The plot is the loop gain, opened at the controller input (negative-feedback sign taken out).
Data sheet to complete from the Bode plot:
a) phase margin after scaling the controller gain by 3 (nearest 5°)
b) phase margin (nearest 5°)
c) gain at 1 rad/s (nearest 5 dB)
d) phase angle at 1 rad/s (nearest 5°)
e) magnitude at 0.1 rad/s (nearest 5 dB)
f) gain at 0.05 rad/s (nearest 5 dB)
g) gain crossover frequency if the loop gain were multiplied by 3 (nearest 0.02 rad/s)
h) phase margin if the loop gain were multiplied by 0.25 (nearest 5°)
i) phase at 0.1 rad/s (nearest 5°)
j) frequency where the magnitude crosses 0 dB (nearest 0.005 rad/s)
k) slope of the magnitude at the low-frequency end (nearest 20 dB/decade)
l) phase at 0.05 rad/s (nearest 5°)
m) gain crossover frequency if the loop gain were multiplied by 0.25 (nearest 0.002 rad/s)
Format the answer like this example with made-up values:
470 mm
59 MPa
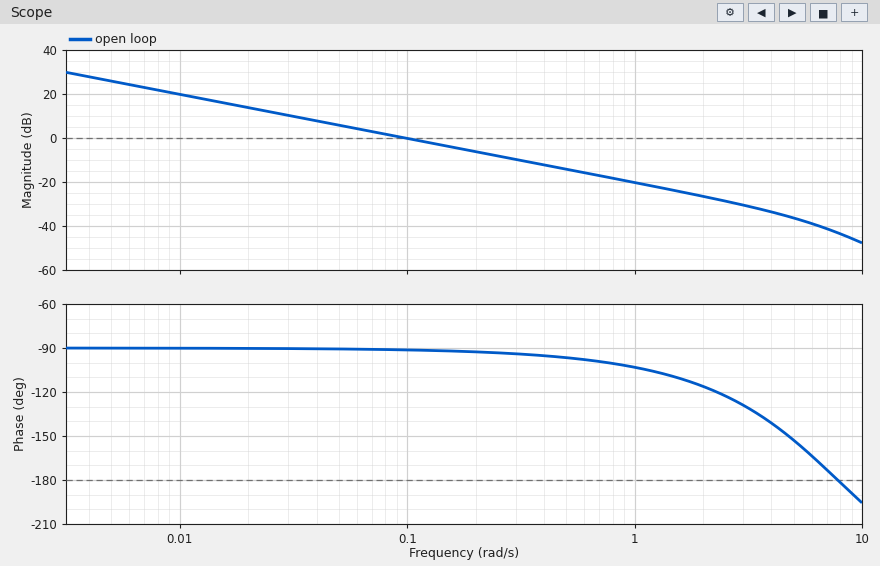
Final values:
85°
90°
-20 dB
-105°
0 dB
5 dB
0.30 rad/s
90°
-90°
0.100 rad/s
-20 dB/decade
-90°
0.024 rad/s
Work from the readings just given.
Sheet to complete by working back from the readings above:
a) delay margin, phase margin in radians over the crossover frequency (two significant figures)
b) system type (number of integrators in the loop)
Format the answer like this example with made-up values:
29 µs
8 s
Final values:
16 s
1
